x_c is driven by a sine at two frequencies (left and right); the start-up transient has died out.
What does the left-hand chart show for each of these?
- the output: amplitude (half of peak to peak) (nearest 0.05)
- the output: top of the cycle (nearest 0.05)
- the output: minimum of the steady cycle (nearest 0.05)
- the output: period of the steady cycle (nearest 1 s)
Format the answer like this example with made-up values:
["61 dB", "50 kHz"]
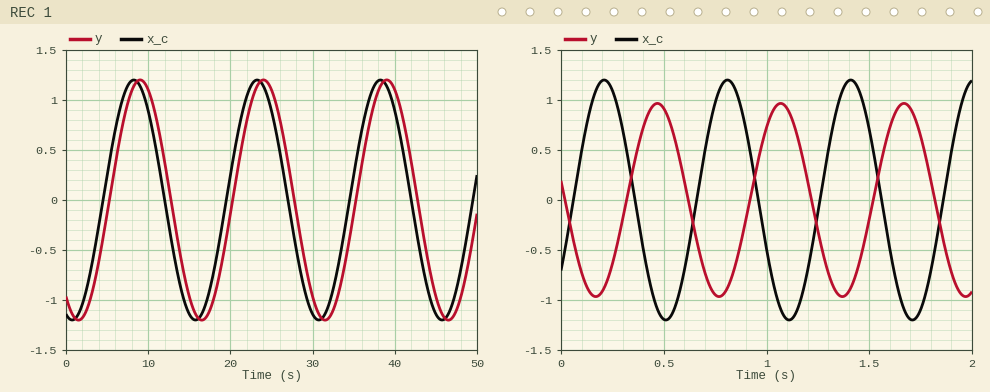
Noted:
["1.20", "1.20", "-1.20", "15 s"]
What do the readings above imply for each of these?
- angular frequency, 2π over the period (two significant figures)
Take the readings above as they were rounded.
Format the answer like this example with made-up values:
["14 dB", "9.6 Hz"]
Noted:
["0.42 rad/s"]
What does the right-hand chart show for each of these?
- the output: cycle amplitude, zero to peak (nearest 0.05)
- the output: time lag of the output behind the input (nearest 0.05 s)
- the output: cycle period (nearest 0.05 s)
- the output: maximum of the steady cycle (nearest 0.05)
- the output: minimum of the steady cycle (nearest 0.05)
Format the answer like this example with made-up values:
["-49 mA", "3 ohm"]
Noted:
["0.95", "0.25 s", "0.60 s", "0.95", "-0.95"]
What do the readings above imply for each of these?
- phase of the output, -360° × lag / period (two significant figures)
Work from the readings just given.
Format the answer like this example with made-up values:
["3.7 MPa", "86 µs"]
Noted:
["-150°"]
